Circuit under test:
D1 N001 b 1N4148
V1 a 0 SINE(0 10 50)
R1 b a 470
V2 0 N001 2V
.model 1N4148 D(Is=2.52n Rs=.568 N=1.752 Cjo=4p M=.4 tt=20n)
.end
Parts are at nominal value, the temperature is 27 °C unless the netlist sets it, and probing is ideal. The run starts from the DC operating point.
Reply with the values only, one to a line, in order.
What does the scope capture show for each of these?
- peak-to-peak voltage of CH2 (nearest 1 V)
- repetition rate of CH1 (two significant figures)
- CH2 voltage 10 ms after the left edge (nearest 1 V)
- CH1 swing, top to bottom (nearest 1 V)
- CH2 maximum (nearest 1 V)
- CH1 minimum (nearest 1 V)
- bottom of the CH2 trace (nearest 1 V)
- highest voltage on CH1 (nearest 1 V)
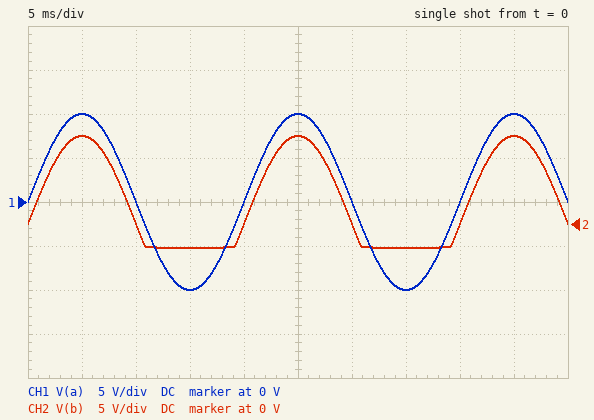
13 V
50 Hz
0 V
20 V
10 V
-10 V
-3 V
10 V
